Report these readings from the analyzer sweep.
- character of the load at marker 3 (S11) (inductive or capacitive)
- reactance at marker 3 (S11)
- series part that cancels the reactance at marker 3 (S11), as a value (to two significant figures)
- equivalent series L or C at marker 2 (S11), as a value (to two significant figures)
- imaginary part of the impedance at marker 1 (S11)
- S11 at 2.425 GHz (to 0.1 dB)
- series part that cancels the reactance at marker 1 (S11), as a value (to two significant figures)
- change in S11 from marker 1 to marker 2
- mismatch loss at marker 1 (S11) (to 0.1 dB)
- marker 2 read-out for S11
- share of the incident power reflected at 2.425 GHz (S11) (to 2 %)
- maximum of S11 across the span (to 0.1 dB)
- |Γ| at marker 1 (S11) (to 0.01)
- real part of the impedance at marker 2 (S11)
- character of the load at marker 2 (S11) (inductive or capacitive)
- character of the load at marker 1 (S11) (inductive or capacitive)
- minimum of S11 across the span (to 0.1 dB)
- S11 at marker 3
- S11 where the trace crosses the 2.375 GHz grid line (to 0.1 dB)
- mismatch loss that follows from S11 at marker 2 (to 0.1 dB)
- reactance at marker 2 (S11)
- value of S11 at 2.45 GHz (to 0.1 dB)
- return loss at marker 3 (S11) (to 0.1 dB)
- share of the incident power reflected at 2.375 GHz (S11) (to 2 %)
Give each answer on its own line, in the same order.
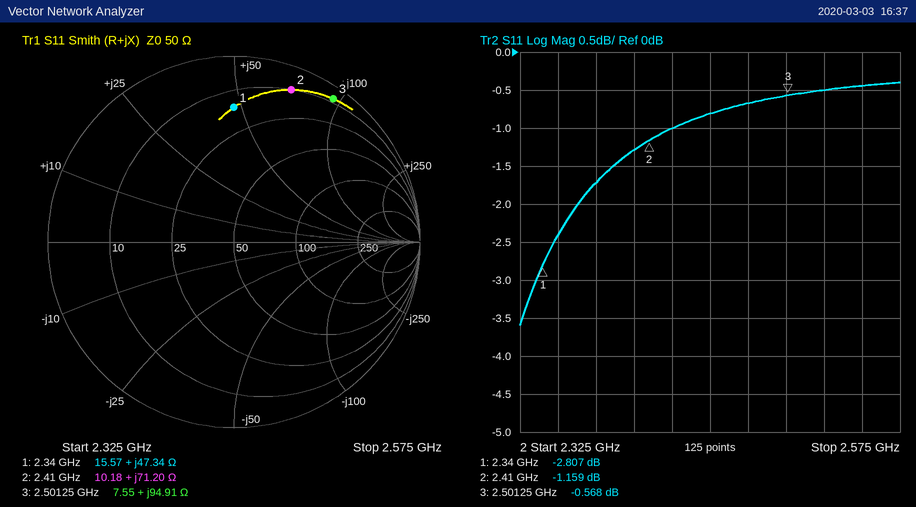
inductive
+94.91 Ω
670 fF
4.7 nH
+47.34 Ω
-1.0 dB
1.4 pF
1.648 dB
3.2 dB
-1.159 dB
80 %
-0.4 dB
0.72
10.18 Ω
inductive
inductive
-3.6 dB
-0.568 dB
-1.7 dB
6.3 dB
+71.20 Ω
-0.8 dB
0.6 dB
68 %
